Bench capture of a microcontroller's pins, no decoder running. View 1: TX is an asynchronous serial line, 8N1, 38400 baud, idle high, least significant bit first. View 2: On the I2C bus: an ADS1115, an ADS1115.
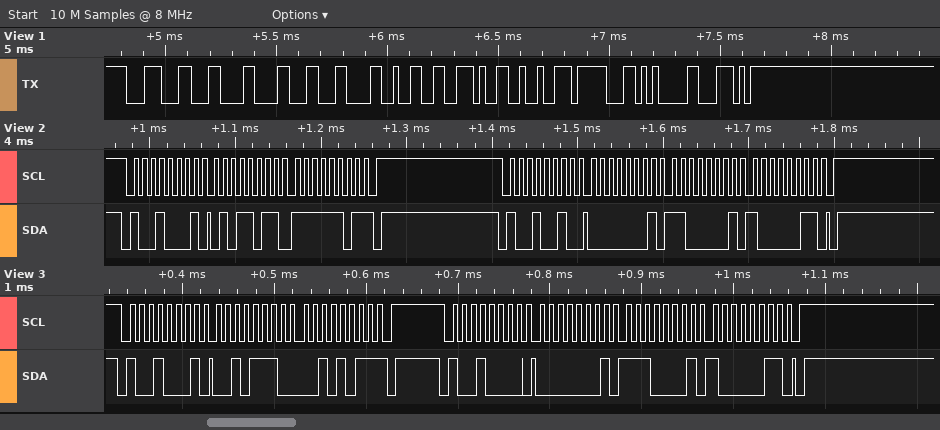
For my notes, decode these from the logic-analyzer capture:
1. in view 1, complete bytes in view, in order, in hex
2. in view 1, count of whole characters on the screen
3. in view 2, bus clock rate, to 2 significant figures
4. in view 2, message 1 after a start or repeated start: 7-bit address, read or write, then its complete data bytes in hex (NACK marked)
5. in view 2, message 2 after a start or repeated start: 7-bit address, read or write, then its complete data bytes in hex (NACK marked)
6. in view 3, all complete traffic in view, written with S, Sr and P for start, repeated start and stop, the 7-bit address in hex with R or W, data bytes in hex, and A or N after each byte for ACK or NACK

1C 0C 18 0C 32 2E 92 1F 05 5C
10
100 kHz
0x48 read: 5B FD NACK
0x49 write: 01 C1 83
S 48R A 2E A 2B N P S 48W A 01 A E1 A 83 A P
